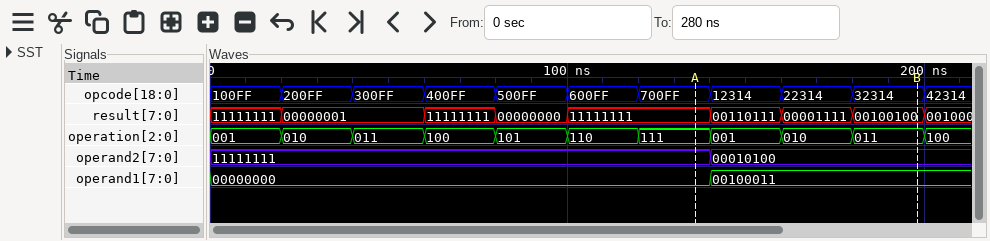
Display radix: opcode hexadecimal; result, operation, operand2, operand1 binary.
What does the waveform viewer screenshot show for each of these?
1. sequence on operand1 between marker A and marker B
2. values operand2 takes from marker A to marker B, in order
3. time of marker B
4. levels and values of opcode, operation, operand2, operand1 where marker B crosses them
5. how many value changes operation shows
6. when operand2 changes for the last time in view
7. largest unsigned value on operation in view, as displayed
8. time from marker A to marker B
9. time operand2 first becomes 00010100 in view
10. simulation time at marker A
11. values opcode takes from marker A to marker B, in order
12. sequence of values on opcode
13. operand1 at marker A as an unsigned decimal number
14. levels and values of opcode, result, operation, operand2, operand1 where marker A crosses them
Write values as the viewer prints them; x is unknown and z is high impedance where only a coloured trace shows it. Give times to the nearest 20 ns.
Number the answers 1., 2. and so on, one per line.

1. 00000000, 00100011
2. 11111111, 00010100
3. 200 ns
4. opcode=32314, operation=011, operand2=00010100, operand1=00100011
5. 10
6. 140 ns
7. 111
8. 60 ns
9. 140 ns
10. 140 ns
11. 700FF, 12314, 22314, 32314
12. 100FF, 200FF, 300FF, 400FF, 500FF, 600FF, 700FF, 12314, 22314, 32314, 42314
13. 0
14. opcode=700FF, result=11111111, operation=111, operand2=11111111, operand1=00000000
